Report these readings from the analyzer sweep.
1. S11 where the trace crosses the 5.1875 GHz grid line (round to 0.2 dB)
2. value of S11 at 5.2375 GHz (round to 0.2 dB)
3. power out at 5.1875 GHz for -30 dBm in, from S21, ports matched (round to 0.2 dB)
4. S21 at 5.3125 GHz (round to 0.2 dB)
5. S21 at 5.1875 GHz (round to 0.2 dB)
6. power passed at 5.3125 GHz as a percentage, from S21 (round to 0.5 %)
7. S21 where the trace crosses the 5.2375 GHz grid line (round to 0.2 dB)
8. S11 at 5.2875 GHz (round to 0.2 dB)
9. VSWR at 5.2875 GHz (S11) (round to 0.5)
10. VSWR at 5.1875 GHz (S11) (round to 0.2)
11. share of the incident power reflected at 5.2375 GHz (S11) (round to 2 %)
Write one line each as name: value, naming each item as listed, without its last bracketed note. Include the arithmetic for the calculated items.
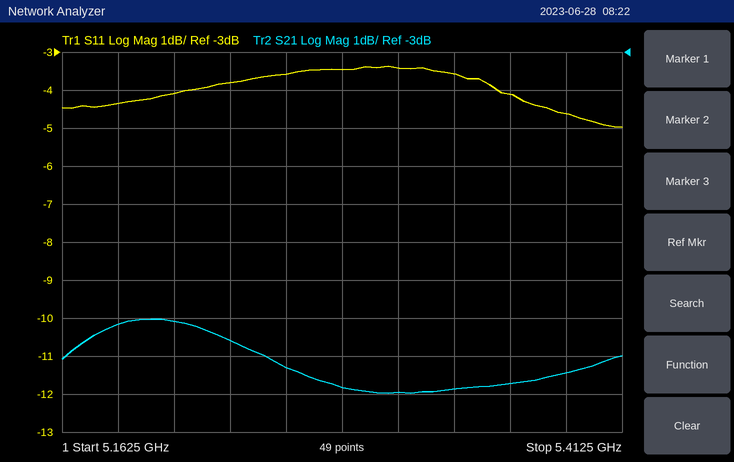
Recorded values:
S11 where the trace crosses the 5.1875 GHz grid line: -4.4 dB
value of S11 at 5.2375 GHz: -3.8 dB
power out at 5.1875 GHz for -30 dBm in, from S21, ports matched: -30 dBm + (-10.2 dB) = -40.2 dBm
S21 at 5.3125 GHz: -12.0 dB
S21 at 5.1875 GHz: -10.2 dB
power passed at 5.3125 GHz as a percentage, from S21: 10^(-12/10) ≈ 6.31 %, so 6.5 % to the nearest 0.5 %
S21 where the trace crosses the 5.2375 GHz grid line: -10.6 dB
S11 at 5.2875 GHz: -3.4 dB
VSWR at 5.2875 GHz (S11): |Γ| = 10^(-3.4/20) = 0.6761; VSWR = (1 + 0.6761)/(1 − 0.6761) ≈ 5.17, so 5.0 to the nearest 0.5
VSWR at 5.1875 GHz (S11): |Γ| = 10^(-4.4/20) = 0.6026; VSWR = (1 + 0.6026)/(1 − 0.6026) ≈ 4.0
share of the incident power reflected at 5.2375 GHz (S11): 10^(-3.8/10) ≈ 42 %
